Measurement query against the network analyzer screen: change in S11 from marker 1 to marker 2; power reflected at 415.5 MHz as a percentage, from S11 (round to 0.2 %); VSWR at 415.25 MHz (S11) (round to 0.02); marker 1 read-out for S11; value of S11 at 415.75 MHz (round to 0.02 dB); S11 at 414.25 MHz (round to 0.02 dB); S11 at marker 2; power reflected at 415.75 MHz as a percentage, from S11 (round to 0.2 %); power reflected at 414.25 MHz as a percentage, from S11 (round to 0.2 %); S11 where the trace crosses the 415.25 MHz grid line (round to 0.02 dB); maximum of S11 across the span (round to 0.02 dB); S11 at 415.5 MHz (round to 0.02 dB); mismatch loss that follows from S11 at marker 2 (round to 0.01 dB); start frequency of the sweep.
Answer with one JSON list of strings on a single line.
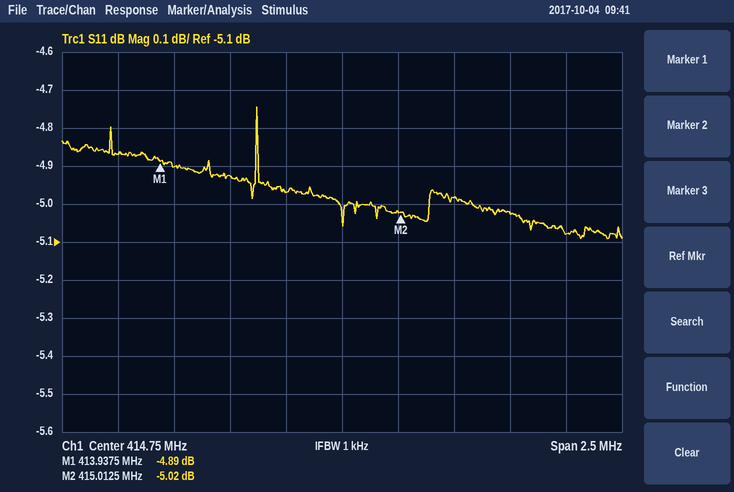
["-0.13 dB", "31.4 %", "3.58", "-4.89 dB", "-5.08 dB", "-4.92 dB", "-5.02 dB", "31.0 %", "32.2 %", "-4.98 dB", "-4.74 dB", "-5.02 dB", "1.64 dB", "413.5 MHz"]
